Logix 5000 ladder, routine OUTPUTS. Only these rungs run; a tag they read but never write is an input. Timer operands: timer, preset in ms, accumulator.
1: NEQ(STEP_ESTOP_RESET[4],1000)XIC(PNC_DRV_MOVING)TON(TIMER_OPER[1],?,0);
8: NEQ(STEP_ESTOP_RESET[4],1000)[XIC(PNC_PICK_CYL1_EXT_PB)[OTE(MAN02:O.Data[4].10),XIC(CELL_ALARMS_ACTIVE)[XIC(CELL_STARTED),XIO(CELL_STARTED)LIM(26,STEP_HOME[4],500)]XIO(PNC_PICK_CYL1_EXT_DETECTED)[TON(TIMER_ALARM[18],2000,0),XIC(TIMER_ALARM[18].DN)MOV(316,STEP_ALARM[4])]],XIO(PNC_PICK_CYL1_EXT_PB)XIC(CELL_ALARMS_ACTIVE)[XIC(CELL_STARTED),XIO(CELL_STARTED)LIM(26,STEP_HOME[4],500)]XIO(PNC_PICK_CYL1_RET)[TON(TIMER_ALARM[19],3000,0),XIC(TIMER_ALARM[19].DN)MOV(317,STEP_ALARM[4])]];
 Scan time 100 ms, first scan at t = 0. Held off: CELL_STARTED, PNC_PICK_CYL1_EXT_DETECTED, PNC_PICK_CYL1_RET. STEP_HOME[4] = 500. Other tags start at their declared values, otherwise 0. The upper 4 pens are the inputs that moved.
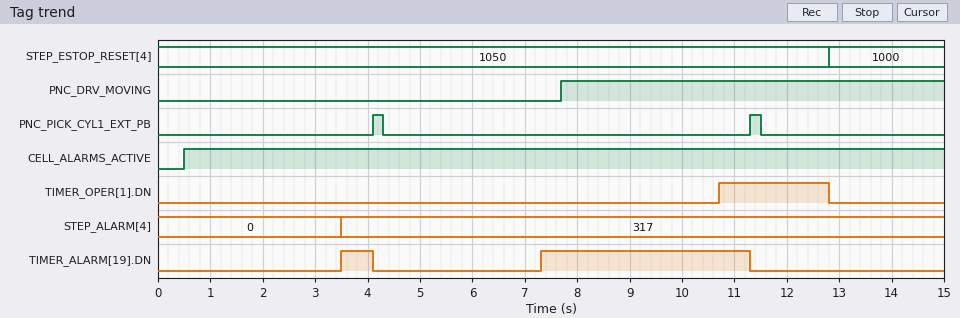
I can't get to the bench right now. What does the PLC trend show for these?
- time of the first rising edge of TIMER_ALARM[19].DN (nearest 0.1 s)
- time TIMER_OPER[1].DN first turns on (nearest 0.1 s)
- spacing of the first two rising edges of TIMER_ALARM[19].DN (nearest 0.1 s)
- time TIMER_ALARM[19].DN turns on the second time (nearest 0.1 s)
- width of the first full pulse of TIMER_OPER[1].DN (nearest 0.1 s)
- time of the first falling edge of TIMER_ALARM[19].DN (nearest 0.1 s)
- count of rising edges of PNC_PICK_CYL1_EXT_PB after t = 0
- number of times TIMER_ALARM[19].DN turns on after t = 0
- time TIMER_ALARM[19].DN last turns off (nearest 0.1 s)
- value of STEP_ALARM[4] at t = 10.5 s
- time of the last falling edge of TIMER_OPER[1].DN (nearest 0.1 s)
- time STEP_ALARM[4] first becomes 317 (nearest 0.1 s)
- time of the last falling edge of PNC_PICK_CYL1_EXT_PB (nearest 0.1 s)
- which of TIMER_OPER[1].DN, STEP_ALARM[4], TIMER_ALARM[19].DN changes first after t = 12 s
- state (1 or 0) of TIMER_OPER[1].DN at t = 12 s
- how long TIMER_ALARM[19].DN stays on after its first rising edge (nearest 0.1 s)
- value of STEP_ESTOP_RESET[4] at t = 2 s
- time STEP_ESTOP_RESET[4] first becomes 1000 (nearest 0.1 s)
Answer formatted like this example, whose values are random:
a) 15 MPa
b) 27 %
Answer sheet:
a) 3.5 s
b) 10.7 s
c) 3.8 s
d) 7.3 s
e) 2.1 s
f) 4.1 s
g) 2
h) 2
i) 11.3 s
j) 317
k) 12.8 s
l) 3.5 s
m) 11.5 s
n) TIMER_OPER[1].DN
o) 1
p) 0.6 s
q) 1050
r) 12.8 s
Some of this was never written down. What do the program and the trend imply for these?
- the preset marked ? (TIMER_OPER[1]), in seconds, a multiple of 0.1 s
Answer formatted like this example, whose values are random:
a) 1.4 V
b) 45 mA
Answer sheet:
a) 3.0 s
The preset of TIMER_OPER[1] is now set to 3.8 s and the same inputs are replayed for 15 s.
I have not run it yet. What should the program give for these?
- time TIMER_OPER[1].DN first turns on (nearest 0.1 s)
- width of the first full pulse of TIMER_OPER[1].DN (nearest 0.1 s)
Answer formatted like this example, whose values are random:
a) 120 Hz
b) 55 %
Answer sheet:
a) 11.5 s
b) 1.3 s
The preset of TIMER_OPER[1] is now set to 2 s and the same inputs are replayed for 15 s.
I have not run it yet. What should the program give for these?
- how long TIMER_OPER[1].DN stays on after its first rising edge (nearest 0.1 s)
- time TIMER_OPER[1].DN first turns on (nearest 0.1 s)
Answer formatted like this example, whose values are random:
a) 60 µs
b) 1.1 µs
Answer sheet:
a) 3.1 s
b) 9.7 s
